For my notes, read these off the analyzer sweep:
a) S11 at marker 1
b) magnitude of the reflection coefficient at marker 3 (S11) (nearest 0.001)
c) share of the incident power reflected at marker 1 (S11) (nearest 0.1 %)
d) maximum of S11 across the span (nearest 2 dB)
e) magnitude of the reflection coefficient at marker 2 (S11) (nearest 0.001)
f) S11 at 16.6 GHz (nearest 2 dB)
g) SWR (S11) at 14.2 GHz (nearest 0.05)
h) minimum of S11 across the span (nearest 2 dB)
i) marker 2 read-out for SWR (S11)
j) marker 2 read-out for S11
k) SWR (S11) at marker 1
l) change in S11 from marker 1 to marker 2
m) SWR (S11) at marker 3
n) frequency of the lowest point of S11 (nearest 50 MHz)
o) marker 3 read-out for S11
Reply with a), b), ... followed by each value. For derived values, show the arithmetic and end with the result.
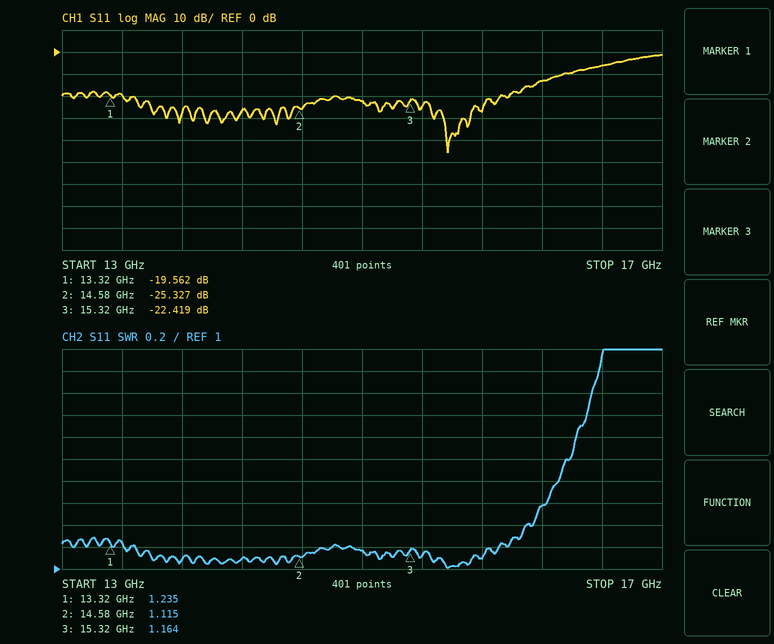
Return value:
a) -19.562 dB
b) 10^(-22.419/20) ≈ 0.076
c) 10^(-19.562/10) ≈ 1.1 %
d) -2 dB
e) 10^(-25.327/20) ≈ 0.054
f) -6 dB
g) 1.10
h) -46 dB
i) 1.115
j) -25.327 dB
k) 1.235
l) -25.327 − (-19.562) = -5.765 dB
m) 1.164
n) 15.55 GHz
o) -22.419 dB
